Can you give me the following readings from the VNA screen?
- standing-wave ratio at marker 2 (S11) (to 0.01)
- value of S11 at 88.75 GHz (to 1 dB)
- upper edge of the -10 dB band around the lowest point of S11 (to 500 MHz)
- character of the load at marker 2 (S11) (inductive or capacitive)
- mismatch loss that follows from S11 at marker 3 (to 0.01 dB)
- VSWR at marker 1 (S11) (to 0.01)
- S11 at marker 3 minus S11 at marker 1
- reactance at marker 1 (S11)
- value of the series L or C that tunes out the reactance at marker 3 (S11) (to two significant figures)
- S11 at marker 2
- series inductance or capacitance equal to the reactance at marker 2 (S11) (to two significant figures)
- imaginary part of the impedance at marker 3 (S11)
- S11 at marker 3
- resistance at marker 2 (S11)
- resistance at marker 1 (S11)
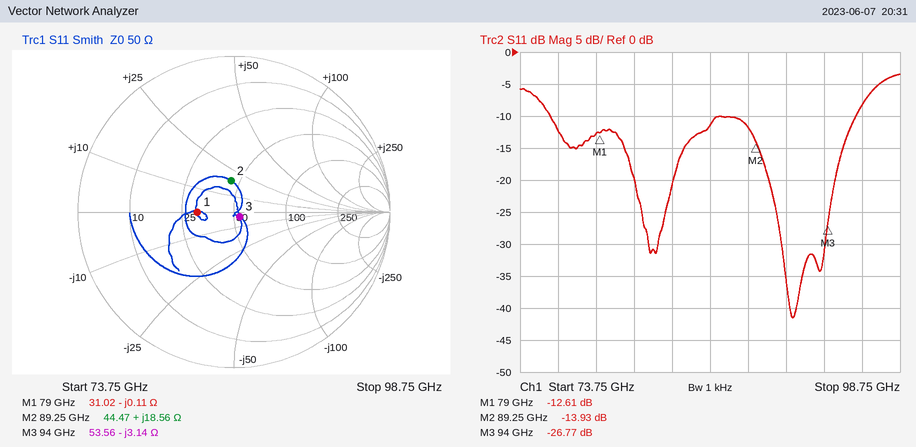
1.50
-12 dB
96.0 GHz
inductive
0.01 dB
1.61
-14.16 dB
-0.11 Ω
5.3 pH
-13.93 dB
33 pH
-3.14 Ω
-26.77 dB
44.47 Ω
31.02 Ω
